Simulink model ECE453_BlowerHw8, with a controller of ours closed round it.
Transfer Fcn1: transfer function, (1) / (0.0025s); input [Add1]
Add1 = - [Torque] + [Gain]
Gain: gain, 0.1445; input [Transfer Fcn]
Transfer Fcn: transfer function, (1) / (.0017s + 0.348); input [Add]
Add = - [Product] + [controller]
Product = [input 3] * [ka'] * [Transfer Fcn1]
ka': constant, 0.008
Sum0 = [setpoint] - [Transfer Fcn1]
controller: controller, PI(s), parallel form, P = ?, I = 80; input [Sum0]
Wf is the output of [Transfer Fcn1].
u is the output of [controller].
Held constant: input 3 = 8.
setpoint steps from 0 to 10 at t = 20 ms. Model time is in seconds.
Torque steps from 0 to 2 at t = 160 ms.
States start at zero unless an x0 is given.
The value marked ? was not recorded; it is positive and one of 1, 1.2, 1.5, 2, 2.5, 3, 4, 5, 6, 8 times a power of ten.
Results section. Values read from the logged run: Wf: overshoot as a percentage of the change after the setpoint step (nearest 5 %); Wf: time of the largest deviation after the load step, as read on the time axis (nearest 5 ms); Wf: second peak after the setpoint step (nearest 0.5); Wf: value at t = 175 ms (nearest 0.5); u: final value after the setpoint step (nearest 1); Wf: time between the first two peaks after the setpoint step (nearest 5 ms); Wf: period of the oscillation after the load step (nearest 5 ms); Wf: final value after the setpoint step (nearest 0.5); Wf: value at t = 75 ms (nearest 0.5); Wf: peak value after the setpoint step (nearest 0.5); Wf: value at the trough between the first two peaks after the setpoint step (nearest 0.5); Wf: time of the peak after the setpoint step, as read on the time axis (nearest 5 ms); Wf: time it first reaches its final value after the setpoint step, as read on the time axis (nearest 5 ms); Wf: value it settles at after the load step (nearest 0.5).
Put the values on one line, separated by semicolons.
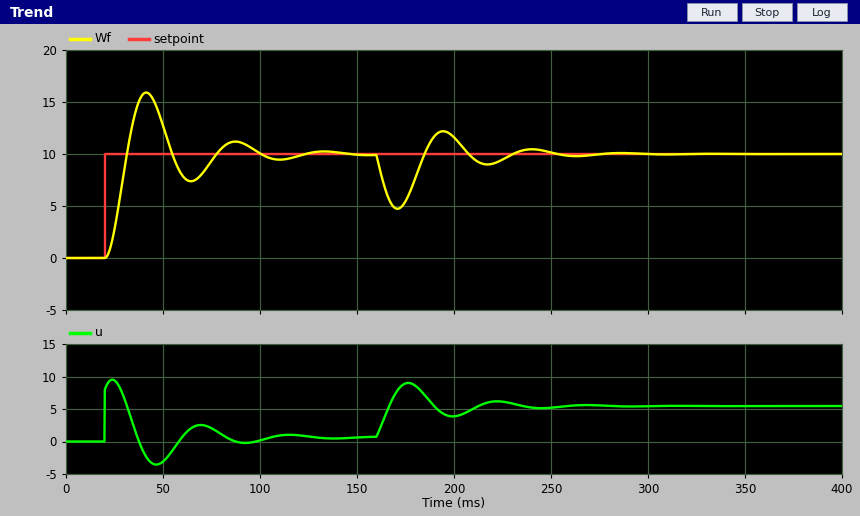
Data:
60 %; 170 ms; 11.0; 5.5; 1; 45 ms; 45 ms; 10.0; 9.5; 16.0; 7.5; 40 ms; 30 ms; 10.0
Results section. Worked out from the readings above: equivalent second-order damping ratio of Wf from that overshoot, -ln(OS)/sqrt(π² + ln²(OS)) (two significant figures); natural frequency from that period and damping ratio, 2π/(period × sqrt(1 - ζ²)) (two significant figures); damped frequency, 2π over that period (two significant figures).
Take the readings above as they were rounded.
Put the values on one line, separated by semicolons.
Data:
0.16; 0.14 rad/ms; 0.14 rad/ms
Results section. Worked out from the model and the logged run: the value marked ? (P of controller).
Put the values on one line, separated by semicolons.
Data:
0.8
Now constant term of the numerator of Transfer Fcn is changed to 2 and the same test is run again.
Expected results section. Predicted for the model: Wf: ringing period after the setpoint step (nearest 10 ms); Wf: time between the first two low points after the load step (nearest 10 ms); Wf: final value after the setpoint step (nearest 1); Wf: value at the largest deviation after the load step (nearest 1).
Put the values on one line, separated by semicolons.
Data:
30 ms; 30 ms; 10; 6
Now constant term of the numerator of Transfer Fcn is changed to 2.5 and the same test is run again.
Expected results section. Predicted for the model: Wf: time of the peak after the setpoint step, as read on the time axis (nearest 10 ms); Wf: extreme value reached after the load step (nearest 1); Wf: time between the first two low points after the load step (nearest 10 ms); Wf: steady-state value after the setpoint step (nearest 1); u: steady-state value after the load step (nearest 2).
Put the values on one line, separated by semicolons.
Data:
30 ms; 7; 30 ms; 10; 2
